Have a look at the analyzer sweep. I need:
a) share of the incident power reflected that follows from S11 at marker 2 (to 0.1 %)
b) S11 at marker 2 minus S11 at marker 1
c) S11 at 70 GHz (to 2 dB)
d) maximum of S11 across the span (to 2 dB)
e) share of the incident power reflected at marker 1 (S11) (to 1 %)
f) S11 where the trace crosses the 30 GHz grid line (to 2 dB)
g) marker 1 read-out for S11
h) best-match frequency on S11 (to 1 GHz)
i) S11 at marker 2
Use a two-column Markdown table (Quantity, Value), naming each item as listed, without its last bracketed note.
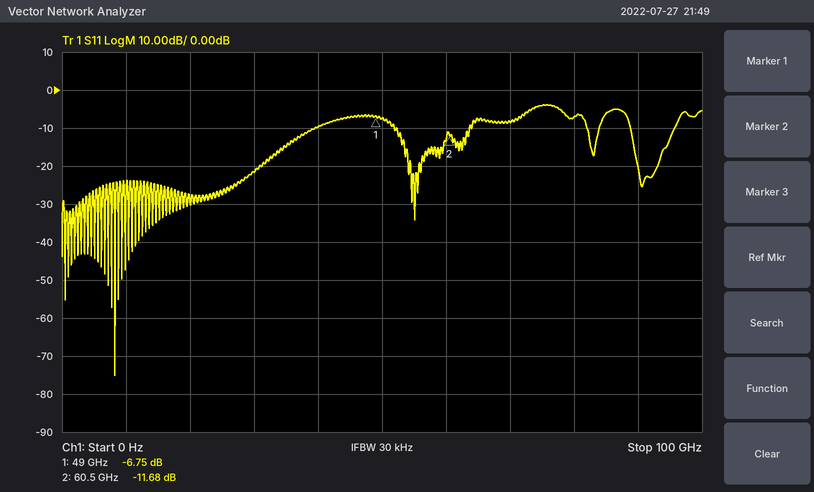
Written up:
| Quantity | Value |
|---|---|
| share of the incident power reflected that follows from S11 at marker 2 | 6.8 % |
| S11 at marker 2 minus S11 at marker 1 | -4.93 dB |
| S11 at 70 GHz | -8 dB |
| maximum of S11 across the span | -4 dB |
| share of the incident power reflected at marker 1 (S11) | 21 % |
| S11 where the trace crosses the 30 GHz grid line | -22 dB |
| marker 1 read-out for S11 | -6.75 dB |
| best-match frequency on S11 | 8 GHz |
| S11 at marker 2 | -11.68 dB |
